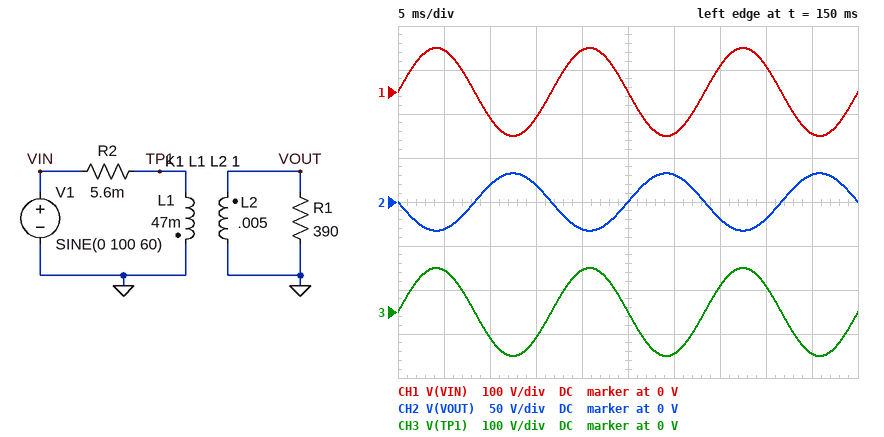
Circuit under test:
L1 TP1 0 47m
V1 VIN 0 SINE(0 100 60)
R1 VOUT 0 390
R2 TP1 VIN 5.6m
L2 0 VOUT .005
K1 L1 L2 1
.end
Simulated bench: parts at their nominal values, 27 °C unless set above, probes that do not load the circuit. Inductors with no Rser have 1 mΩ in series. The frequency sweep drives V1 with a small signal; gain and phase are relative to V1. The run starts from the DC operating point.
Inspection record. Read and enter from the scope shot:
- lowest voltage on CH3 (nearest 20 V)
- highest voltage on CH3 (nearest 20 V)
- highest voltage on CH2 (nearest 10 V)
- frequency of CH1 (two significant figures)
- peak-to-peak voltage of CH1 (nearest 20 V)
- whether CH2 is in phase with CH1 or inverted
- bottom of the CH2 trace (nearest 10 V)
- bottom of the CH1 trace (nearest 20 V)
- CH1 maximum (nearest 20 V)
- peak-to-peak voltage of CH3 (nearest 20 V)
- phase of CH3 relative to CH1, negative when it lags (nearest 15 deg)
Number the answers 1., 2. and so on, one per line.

1. -100 V
2. 100 V
3. 30 V
4. 60 Hz
5. 200 V
6. inverted
7. -30 V
8. -100 V
9. 100 V
10. 200 V
11. 0 deg
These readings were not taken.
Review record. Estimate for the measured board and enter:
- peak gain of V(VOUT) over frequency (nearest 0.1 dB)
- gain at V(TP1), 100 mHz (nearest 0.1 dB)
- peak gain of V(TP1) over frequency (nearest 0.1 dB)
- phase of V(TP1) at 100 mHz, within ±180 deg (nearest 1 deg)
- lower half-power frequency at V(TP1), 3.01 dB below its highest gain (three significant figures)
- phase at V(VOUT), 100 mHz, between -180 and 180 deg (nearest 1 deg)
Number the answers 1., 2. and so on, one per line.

1. -9.7 dB
2. -0.2 dB
3. 0 dB
4. 11 deg
5. 21.8 mHz
6. -167 deg
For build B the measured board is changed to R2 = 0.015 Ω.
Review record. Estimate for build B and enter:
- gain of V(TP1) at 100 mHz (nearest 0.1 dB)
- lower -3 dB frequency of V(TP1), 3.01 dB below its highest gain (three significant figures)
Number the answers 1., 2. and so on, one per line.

1. -1.1 dB
2. 54.0 mHz
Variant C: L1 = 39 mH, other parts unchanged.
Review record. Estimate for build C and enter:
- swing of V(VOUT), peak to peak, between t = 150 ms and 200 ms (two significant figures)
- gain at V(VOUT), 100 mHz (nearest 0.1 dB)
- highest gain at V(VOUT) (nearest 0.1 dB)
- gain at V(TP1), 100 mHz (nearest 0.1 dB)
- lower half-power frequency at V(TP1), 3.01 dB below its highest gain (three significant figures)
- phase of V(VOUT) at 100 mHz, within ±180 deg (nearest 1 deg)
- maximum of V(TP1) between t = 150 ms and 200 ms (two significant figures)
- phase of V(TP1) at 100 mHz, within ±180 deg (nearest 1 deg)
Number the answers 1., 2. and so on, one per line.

1. 72 V
2. -9.2 dB
3. -8.9 dB
4. -0.3 dB
5. 26.3 mHz
6. -165 deg
7. 100 V
8. 13 deg
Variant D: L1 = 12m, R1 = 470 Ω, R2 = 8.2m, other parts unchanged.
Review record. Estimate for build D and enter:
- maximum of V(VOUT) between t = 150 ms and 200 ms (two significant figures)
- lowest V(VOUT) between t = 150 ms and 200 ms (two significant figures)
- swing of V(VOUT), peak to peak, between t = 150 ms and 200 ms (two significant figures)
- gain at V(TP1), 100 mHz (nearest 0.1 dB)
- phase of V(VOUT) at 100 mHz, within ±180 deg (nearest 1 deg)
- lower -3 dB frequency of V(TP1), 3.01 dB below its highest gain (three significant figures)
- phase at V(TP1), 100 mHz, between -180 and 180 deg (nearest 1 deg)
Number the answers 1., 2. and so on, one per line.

1. 65 V
2. -64 V
3. 130 V
4. -3.9 dB
5. -129 deg
6. 121 mHz
7. 43 deg
